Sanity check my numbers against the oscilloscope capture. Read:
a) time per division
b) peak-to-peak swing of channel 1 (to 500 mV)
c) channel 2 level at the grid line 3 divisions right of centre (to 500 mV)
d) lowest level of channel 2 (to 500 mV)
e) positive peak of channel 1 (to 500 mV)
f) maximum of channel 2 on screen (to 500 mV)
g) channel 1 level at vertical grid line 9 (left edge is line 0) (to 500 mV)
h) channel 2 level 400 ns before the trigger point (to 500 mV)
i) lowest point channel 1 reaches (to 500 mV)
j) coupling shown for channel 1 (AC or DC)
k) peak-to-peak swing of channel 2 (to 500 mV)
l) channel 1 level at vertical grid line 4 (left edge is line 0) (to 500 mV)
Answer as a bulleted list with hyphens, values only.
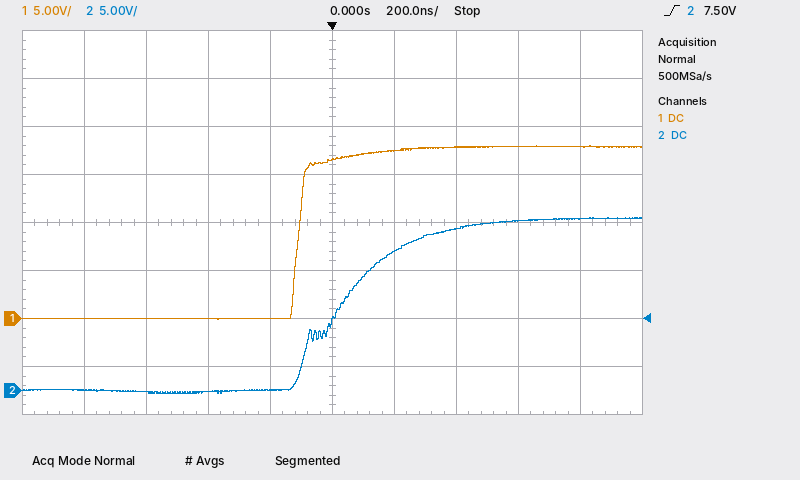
- 200 ns
- 18.0 V
- 17.5 V
- -500 mV
- 18.0 V
- 18.0 V
- 18.0 V
- 0.0 V
- 0.0 V
- DC
- 18.5 V
- 0.0 V
